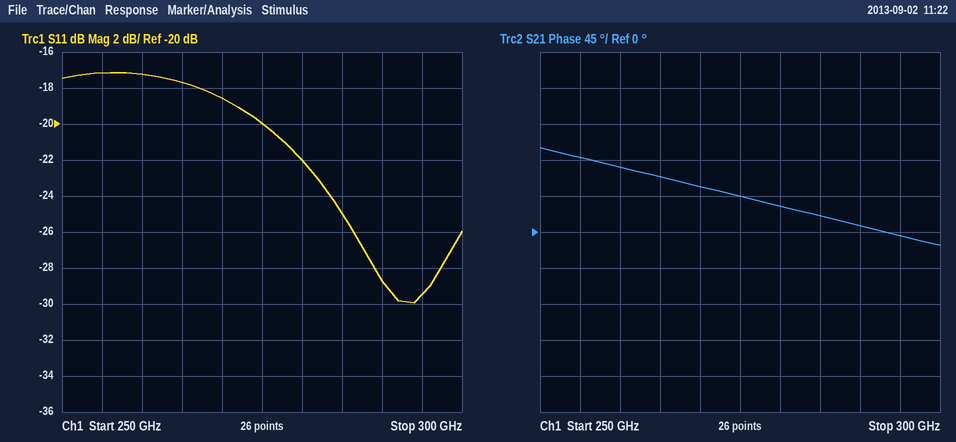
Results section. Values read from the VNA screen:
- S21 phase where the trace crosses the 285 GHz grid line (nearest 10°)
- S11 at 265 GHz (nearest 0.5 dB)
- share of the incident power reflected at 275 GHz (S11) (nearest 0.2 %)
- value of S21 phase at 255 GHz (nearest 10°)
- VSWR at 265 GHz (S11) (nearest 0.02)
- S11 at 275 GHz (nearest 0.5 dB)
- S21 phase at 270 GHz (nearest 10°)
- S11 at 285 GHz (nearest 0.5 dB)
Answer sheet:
20°
-17.5 dB
1.0 %
90°
1.30
-20.0 dB
60°
-25.0 dB
